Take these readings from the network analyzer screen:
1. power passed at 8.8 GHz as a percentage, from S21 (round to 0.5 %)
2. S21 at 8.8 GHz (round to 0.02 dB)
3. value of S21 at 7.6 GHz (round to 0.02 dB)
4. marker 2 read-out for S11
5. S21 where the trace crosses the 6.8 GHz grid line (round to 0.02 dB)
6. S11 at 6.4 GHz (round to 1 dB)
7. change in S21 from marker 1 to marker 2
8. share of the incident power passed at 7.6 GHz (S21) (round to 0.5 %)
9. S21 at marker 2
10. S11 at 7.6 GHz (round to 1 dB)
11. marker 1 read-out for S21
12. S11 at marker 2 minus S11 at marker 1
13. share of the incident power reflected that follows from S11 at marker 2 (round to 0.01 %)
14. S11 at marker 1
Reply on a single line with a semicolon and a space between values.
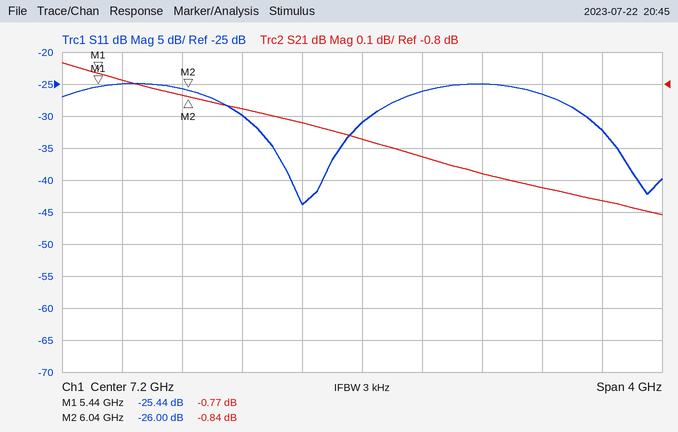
76.5 %; -1.16 dB; -1.02 dB; -26.00 dB; -0.92 dB; -30 dB; -0.07 dB; 79.0 %; -0.84 dB; -26 dB; -0.77 dB; -0.56 dB; 0.25 %; -25.44 dB
